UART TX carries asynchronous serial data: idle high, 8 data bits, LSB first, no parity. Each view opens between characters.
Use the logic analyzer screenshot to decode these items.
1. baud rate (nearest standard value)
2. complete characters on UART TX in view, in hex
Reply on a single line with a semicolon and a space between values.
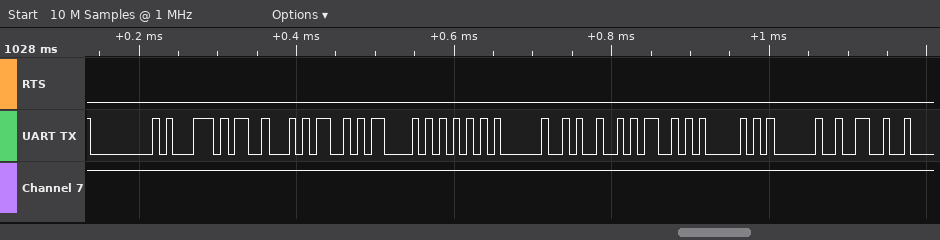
115200 baud; 00, 71, 13, 4D, 43, 55, 20, 49, 53, 50, 20, 26
